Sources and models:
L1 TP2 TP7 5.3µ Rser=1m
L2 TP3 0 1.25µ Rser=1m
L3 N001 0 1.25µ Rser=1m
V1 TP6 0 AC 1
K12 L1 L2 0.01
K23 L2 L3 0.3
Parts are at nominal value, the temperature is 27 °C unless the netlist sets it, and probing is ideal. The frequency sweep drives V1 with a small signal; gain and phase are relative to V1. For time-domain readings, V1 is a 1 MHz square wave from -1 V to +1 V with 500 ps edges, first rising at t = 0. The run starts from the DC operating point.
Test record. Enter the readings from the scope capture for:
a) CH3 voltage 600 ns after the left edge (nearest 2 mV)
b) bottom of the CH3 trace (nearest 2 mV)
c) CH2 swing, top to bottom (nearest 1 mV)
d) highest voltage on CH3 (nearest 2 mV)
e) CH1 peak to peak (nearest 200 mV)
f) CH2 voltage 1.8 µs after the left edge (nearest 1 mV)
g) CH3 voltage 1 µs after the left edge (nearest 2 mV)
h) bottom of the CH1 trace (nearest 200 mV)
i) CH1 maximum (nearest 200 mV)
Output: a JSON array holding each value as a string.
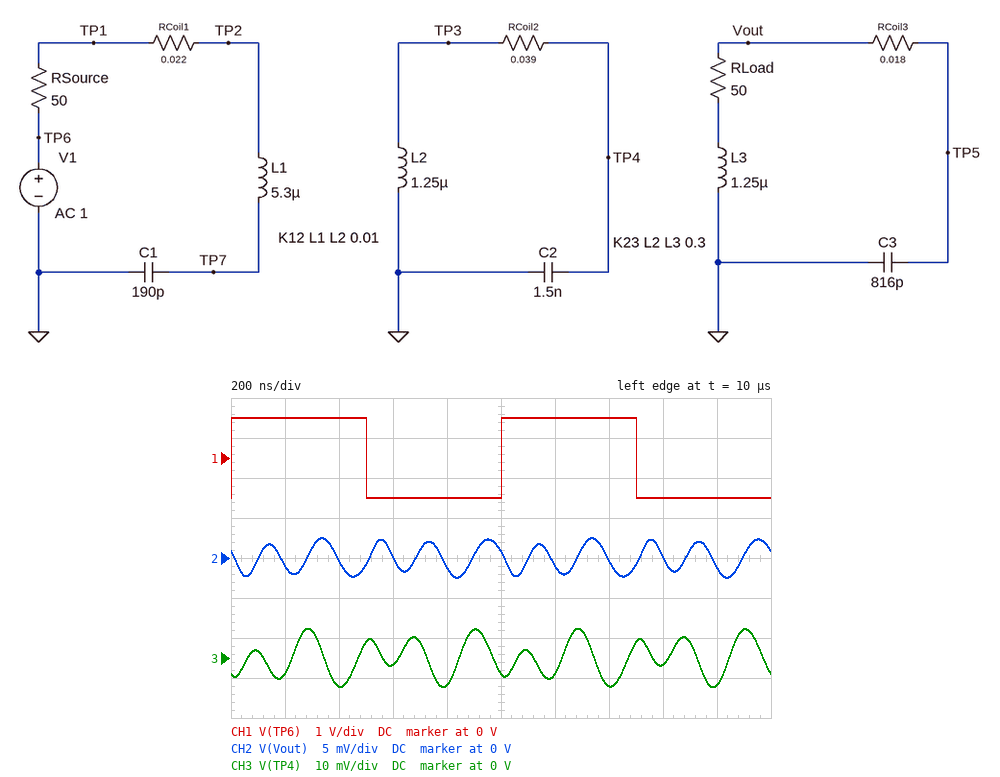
["-2 mV", "-8 mV", "5 mV", "8 mV", "2.0 V", "-1 mV", "-4 mV", "-1.0 V", "1.0 V"]
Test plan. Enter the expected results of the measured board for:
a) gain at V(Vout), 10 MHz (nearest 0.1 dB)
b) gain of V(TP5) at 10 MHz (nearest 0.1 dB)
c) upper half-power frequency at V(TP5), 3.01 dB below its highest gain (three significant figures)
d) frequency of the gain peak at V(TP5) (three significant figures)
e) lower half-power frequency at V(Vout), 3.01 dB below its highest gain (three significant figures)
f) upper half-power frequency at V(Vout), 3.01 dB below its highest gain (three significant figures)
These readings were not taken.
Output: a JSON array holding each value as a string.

["-64.4 dB", "-64.4 dB", "3.73 MHz", "3.64 MHz", "3.57 MHz", "3.73 MHz"]
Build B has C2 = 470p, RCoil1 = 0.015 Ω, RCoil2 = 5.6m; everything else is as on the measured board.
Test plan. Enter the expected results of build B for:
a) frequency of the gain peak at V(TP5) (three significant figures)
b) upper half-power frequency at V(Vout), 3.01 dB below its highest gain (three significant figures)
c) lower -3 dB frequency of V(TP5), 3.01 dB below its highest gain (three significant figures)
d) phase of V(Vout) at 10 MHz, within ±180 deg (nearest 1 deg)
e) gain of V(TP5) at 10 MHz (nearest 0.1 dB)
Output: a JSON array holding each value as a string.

["6.65 MHz", "6.92 MHz", "6.33 MHz", "58 deg", "-60.4 dB"]
